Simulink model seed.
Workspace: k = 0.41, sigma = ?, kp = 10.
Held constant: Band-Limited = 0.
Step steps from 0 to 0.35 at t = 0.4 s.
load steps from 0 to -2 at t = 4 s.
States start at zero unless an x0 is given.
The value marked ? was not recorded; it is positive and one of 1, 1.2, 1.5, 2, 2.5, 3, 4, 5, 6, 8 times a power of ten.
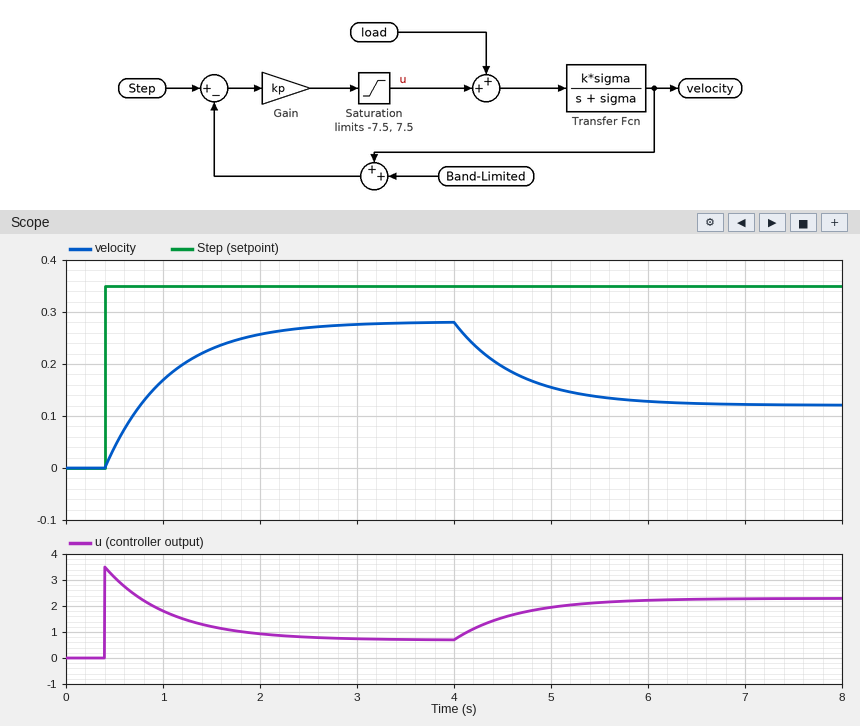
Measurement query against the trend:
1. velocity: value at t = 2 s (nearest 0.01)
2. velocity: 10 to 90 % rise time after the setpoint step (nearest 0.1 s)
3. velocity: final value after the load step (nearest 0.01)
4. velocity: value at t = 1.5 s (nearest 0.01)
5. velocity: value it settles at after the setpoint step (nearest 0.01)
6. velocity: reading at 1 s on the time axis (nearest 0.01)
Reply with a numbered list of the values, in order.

1. 0.26
2. 1.4 s
3. 0.12
4. 0.23
5. 0.28
6. 0.17
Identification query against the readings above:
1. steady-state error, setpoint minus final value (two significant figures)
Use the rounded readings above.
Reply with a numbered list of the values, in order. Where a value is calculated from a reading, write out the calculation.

1. 0.35 - 0.28 = 0.070
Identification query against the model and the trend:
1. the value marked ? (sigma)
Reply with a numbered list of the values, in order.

1. 0.3
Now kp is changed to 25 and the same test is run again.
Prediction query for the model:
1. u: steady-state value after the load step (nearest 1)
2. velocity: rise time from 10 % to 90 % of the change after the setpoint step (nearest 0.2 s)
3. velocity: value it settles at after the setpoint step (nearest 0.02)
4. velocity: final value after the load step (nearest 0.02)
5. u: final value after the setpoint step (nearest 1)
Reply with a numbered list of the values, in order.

1. 3
2. 0.6 s
3. 0.32
4. 0.24
5. 1
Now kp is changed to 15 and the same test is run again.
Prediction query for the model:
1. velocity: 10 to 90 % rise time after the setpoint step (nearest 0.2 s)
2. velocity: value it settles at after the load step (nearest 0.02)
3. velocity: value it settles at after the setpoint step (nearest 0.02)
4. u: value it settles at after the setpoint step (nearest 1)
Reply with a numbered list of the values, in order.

1. 1.0 s
2. 0.18
3. 0.30
4. 1
